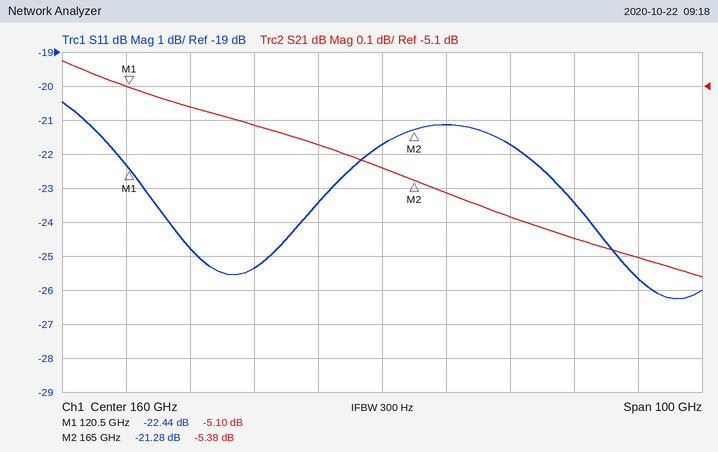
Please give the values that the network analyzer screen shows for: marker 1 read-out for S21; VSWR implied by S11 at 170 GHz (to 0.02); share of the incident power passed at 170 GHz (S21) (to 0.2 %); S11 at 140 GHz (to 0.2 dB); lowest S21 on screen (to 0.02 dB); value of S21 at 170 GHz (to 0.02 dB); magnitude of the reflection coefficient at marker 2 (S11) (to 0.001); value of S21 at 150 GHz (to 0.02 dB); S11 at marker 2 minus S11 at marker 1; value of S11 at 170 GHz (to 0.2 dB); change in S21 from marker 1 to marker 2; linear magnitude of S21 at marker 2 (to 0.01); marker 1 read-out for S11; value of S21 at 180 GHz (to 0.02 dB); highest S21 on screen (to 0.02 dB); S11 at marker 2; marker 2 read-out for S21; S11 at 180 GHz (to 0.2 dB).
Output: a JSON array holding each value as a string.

["-5.10 dB", "1.20", "28.8 %", "-25.4 dB", "-5.66 dB", "-5.42 dB", "0.086", "-5.28 dB", "1.16 dB", "-21.2 dB", "-0.28 dB", "0.54", "-22.44 dB", "-5.48 dB", "-5.02 dB", "-21.28 dB", "-5.38 dB", "-21.8 dB"]
